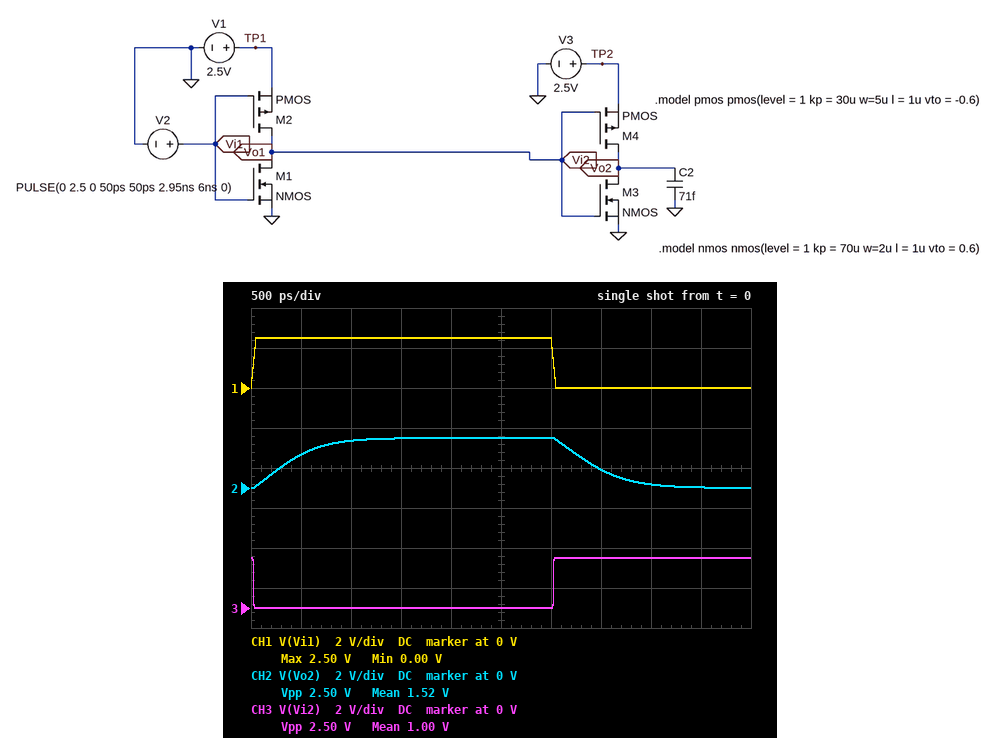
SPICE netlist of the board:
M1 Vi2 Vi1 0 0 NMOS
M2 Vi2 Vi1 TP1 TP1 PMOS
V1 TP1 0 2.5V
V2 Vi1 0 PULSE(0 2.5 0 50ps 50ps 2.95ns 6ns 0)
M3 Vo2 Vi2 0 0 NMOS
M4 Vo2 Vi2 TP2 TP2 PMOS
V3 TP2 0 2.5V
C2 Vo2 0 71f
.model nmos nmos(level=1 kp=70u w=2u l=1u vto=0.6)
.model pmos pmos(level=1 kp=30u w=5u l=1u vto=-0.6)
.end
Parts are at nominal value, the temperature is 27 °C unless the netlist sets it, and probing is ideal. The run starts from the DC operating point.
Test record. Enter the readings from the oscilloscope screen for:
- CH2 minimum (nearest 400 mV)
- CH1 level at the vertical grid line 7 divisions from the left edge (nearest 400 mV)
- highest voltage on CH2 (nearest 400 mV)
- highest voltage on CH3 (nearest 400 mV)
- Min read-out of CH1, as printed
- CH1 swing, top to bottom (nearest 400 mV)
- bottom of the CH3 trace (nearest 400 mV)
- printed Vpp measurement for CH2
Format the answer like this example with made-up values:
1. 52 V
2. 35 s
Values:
1. 0 V
2. 0 V
3. 2.4 V
4. 2.4 V
5. 0.00 V
6. 2.4 V
7. 0 V
8. 2.50 V
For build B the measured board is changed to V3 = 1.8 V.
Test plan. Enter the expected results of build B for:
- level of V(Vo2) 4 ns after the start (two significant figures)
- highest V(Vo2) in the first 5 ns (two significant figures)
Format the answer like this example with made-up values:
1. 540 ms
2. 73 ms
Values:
1. 87 mV
2. 1.8 V
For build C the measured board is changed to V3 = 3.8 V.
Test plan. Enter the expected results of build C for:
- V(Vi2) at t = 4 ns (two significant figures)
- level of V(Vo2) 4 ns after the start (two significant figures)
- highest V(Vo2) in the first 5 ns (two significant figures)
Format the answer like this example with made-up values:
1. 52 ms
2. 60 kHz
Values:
1. 2.5 V
2. 930 mV
3. 3.8 V
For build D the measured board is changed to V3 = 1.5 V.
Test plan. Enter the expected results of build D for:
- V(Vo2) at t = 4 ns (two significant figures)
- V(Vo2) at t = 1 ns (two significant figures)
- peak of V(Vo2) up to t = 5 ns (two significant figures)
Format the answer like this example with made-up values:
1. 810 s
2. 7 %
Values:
1. 62 mV
2. 830 mV
3. 1.5 V
